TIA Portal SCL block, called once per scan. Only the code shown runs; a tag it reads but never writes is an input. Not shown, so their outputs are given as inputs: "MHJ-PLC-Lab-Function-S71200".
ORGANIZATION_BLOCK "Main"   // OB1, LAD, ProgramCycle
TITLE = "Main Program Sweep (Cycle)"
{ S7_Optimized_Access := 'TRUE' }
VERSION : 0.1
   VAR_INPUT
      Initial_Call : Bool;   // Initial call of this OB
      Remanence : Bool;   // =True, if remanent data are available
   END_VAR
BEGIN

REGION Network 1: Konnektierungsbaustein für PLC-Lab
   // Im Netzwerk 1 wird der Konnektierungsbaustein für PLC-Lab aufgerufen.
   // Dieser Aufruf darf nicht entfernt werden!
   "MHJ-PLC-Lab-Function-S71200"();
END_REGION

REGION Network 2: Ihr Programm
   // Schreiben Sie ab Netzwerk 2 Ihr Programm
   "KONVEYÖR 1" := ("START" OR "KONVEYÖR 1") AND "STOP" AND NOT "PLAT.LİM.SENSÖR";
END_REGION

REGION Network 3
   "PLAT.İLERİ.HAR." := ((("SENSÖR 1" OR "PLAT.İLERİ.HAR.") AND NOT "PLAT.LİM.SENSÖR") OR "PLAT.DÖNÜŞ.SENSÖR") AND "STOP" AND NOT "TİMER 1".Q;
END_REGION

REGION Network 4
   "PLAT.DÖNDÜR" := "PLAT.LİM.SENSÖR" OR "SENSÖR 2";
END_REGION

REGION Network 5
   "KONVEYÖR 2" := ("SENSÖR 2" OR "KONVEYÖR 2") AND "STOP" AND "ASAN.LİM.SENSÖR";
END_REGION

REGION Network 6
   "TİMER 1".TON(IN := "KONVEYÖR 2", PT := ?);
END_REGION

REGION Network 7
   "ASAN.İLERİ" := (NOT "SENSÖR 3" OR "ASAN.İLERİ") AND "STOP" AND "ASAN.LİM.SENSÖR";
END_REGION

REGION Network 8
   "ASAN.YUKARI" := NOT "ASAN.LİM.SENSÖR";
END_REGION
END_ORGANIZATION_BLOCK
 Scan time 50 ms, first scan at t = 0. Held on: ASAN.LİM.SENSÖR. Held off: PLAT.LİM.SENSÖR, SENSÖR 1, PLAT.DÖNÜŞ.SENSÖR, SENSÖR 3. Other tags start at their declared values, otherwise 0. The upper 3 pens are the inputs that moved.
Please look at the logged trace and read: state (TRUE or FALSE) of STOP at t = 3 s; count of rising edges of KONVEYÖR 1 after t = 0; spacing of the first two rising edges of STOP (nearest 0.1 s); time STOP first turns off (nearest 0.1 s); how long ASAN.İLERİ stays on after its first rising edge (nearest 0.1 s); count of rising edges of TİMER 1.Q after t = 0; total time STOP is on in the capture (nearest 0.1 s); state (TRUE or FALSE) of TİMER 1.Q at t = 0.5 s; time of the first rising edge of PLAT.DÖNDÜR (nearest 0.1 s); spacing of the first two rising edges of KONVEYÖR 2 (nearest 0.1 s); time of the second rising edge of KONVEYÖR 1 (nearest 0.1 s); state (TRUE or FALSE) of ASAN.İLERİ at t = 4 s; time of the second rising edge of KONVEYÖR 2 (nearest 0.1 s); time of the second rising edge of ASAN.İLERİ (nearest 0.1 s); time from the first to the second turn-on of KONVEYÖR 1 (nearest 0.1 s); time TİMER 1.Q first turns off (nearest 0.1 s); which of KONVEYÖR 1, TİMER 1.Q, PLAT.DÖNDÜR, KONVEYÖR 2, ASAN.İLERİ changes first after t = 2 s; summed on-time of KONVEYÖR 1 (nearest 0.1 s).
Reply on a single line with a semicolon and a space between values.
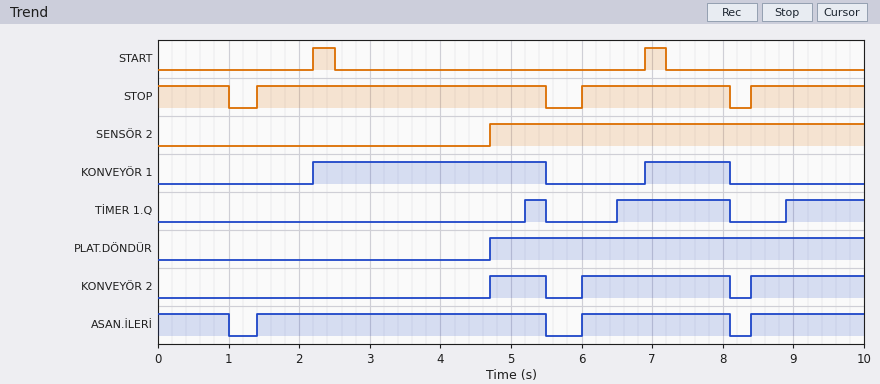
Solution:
TRUE; 2; 4.6 s; 1.0 s; 4.1 s; 3; 8.8 s; FALSE; 4.7 s; 1.3 s; 6.9 s; TRUE; 6.0 s; 6.0 s; 4.7 s; 5.5 s; KONVEYÖR 1; 4.5 s
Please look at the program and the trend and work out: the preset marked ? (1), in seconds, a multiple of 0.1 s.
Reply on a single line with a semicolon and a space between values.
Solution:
0.5 s
